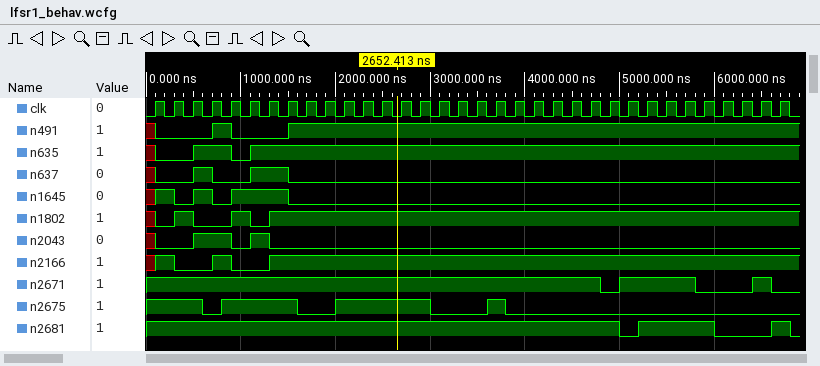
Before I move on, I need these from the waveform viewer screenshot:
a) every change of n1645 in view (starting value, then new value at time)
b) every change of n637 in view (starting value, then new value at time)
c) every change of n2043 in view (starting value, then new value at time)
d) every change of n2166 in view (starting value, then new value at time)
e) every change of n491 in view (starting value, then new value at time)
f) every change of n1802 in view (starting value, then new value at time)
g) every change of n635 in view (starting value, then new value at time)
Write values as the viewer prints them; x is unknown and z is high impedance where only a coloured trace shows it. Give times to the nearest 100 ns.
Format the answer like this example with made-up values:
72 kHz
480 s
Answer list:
x, 1 at 100 ns, 0 at 300 ns, 1 at 500 ns, 0 at 700 ns, 1 at 900 ns, 0 at 1500 ns
x, 0 at 100 ns, 1 at 500 ns, 0 at 700 ns, 1 at 1100 ns, 0 at 1500 ns
x, 0 at 100 ns, 1 at 500 ns, 0 at 900 ns, 1 at 1100 ns, 0 at 1300 ns
x, 1 at 100 ns, 0 at 300 ns, 1 at 700 ns, 0 at 900 ns, 1 at 1300 ns
x, 0 at 100 ns, 1 at 700 ns, 0 at 900 ns, 1 at 1500 ns
x, 0 at 100 ns, 1 at 300 ns, 0 at 500 ns, 1 at 900 ns, 0 at 1100 ns, 1 at 1300 ns
x, 0 at 100 ns, 1 at 500 ns, 0 at 900 ns, 1 at 1100 ns
